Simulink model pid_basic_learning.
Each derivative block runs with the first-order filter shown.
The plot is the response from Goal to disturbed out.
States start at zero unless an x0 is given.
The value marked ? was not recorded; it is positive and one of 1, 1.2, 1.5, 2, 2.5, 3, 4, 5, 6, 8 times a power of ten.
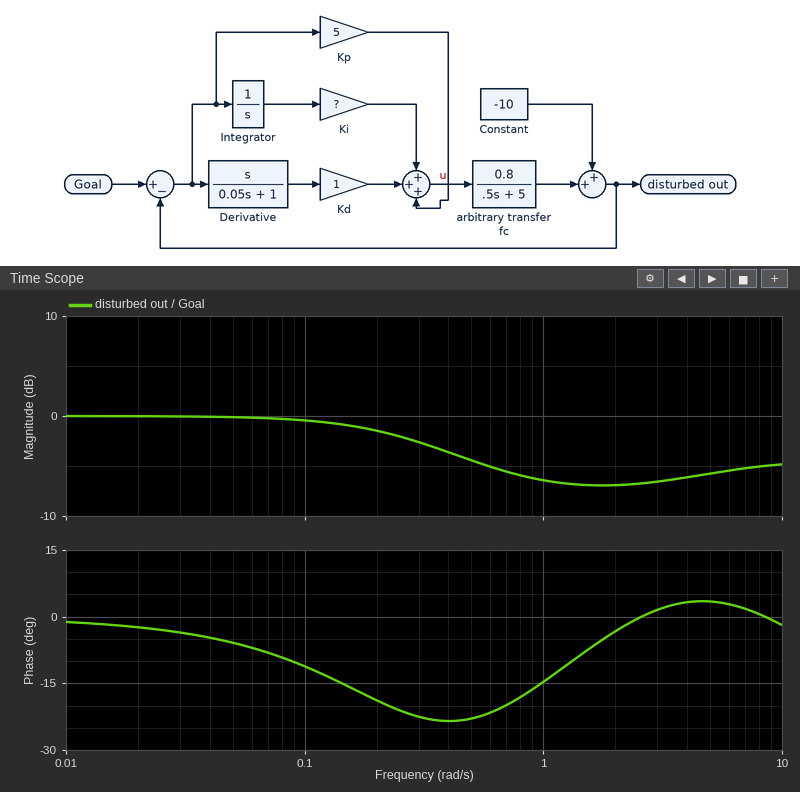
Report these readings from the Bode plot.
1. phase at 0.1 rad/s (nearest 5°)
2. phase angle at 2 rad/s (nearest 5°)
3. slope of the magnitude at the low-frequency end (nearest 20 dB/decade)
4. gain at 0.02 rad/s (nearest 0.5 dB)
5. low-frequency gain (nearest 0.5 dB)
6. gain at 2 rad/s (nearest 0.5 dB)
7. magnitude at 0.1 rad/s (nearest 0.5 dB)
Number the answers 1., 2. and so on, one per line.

1. -10°
2. -5°
3. 0 dB/decade
4. 0.0 dB
5. 0.0 dB
6. -7.0 dB
7. -0.5 dB
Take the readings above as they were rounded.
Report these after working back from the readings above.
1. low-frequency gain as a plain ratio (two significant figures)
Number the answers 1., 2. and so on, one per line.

1. 1.0
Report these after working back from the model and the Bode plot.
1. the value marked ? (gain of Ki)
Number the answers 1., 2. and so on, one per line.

1. 3
